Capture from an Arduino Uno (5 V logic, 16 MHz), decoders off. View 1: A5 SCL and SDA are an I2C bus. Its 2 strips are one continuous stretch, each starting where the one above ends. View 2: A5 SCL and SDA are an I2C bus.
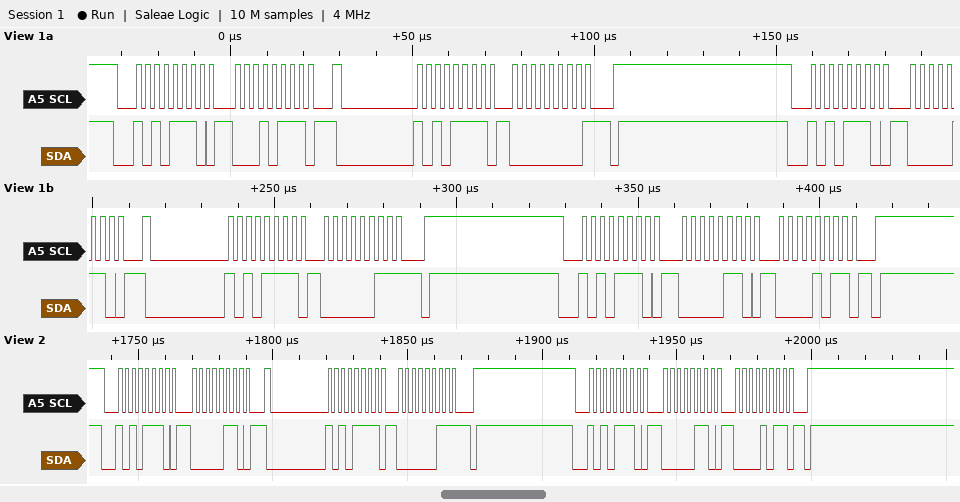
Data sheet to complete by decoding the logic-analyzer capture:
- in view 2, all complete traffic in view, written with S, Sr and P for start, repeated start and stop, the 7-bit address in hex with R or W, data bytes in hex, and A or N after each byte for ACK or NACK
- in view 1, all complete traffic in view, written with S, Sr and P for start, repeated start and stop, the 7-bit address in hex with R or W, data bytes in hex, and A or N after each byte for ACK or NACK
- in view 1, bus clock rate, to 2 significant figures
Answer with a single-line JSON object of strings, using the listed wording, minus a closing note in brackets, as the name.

{"in view 2, all complete traffic in view, written with S, Sr and P for start, repeated start and stop, the 7-bit address in hex with R or W, data bytes in hex, and A or N after each byte for ACK or NACK": "S 57W A 06 A Sr 57R A 03 N P S 57W A 06 A 0B A P", "in view 1, all complete traffic in view, written with S, Sr and P for start, repeated start and stop, the 7-bit address in hex with R or W, data bytes in hex, and A or N after each byte for ACK or NACK": "S 57W A 17 A Sr 57R A 00 N P S 57W A 06 A Sr 57R A 03 N P S 57W A 06 A 0B A P", "in view 1, bus clock rate, to 2 significant figures": "400 kHz"}
